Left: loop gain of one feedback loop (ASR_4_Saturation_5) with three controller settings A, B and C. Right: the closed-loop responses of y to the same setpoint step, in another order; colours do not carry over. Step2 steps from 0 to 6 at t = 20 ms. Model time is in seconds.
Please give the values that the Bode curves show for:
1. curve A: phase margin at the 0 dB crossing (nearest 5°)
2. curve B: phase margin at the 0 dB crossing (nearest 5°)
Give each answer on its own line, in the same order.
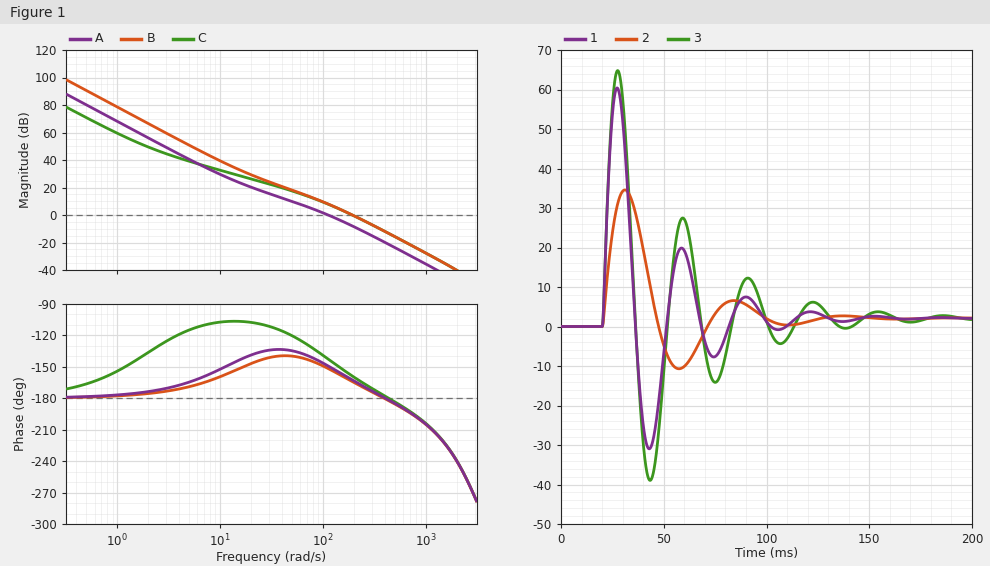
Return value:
30°
15°
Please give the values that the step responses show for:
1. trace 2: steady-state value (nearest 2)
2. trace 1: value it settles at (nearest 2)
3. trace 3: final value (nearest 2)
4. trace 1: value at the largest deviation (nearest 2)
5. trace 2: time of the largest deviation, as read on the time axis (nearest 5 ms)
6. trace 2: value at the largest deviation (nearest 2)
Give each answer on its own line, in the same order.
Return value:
2
2
2
60
30 ms
34
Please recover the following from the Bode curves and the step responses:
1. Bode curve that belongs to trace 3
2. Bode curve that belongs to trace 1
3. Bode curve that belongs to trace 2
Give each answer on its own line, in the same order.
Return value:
B
C
A
